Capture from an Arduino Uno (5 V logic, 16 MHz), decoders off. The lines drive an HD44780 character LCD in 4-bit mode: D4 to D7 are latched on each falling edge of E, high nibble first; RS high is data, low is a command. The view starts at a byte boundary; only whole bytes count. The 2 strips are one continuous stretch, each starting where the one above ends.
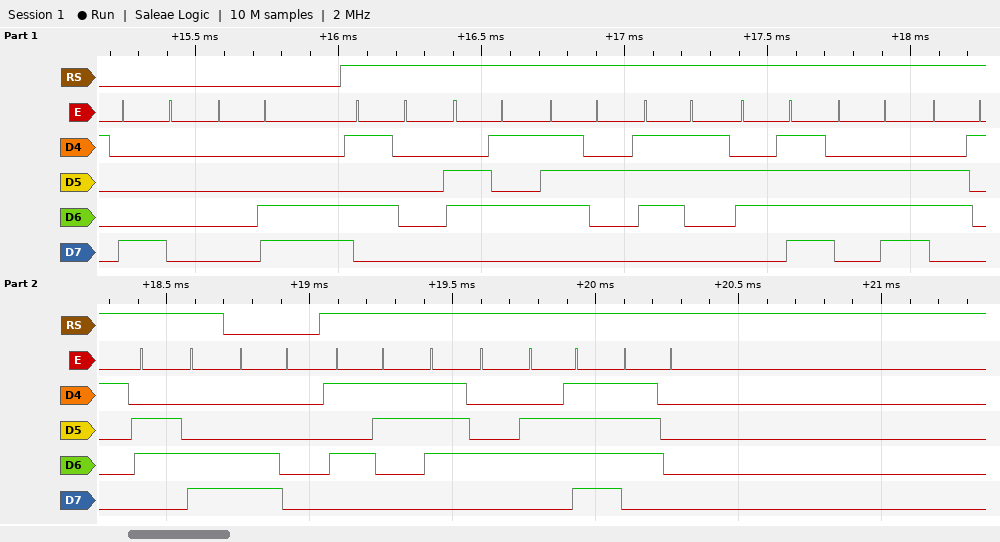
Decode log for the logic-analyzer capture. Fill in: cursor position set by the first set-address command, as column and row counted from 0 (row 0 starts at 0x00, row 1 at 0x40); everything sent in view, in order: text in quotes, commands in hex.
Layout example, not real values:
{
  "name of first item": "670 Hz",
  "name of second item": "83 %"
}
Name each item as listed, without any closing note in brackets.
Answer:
{
  "cursor position set by the first set-address command, as column and row counted from 0": "column 0, row 0",
  "everything sent in view, in order: text in quotes, commands in hex": "0x80 0x0C \"Personal\" 0xC0 \"Stop\""
}
